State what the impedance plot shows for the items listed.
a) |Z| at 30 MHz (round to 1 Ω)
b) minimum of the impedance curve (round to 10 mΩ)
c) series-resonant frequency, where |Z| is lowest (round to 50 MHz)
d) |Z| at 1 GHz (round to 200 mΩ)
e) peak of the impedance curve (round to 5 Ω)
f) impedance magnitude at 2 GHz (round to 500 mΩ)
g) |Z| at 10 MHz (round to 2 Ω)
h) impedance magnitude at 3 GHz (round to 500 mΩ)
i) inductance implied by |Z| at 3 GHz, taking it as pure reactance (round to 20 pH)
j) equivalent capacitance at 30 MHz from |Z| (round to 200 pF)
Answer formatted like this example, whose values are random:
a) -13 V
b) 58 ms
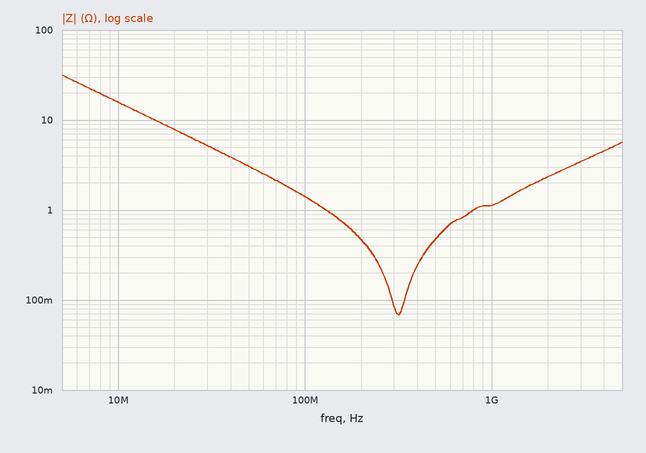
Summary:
a) 5 Ω
b) 70 mΩ
c) 300 MHz
d) 1.2 Ω
e) 30 Ω
f) 2.5 Ω
g) 16 Ω
h) 3.5 Ω
i) 180 pH
j) 1.0 nF
